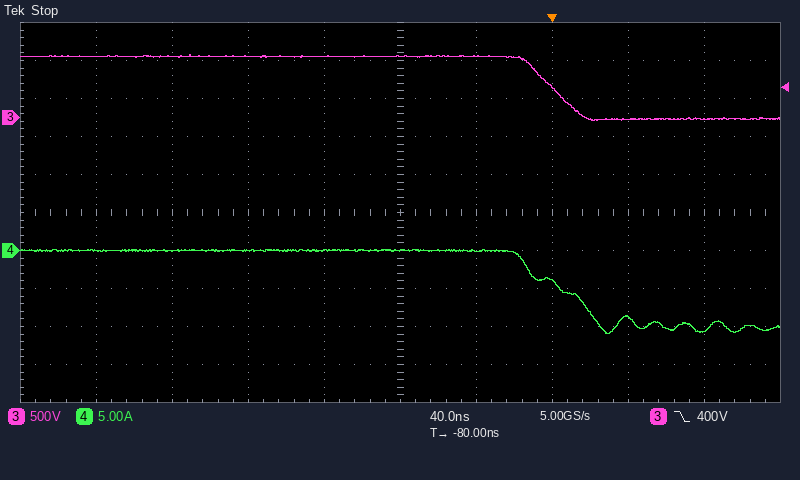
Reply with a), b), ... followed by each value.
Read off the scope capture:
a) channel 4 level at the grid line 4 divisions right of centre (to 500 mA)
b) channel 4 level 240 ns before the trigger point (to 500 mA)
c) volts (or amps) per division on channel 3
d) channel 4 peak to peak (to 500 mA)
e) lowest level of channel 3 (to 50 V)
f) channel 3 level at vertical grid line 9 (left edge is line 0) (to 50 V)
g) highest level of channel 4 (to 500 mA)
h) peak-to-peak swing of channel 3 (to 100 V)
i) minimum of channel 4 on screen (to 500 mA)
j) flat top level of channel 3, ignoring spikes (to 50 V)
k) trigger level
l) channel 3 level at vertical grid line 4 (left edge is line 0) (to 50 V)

a) -10.5 A
b) 0.0 A
c) 500 V
d) 11.0 A
e) -50 V
f) 0 V
g) 0.0 A
h) 900 V
i) -11.0 A
j) 800 V
k) 400 V
l) 800 V
